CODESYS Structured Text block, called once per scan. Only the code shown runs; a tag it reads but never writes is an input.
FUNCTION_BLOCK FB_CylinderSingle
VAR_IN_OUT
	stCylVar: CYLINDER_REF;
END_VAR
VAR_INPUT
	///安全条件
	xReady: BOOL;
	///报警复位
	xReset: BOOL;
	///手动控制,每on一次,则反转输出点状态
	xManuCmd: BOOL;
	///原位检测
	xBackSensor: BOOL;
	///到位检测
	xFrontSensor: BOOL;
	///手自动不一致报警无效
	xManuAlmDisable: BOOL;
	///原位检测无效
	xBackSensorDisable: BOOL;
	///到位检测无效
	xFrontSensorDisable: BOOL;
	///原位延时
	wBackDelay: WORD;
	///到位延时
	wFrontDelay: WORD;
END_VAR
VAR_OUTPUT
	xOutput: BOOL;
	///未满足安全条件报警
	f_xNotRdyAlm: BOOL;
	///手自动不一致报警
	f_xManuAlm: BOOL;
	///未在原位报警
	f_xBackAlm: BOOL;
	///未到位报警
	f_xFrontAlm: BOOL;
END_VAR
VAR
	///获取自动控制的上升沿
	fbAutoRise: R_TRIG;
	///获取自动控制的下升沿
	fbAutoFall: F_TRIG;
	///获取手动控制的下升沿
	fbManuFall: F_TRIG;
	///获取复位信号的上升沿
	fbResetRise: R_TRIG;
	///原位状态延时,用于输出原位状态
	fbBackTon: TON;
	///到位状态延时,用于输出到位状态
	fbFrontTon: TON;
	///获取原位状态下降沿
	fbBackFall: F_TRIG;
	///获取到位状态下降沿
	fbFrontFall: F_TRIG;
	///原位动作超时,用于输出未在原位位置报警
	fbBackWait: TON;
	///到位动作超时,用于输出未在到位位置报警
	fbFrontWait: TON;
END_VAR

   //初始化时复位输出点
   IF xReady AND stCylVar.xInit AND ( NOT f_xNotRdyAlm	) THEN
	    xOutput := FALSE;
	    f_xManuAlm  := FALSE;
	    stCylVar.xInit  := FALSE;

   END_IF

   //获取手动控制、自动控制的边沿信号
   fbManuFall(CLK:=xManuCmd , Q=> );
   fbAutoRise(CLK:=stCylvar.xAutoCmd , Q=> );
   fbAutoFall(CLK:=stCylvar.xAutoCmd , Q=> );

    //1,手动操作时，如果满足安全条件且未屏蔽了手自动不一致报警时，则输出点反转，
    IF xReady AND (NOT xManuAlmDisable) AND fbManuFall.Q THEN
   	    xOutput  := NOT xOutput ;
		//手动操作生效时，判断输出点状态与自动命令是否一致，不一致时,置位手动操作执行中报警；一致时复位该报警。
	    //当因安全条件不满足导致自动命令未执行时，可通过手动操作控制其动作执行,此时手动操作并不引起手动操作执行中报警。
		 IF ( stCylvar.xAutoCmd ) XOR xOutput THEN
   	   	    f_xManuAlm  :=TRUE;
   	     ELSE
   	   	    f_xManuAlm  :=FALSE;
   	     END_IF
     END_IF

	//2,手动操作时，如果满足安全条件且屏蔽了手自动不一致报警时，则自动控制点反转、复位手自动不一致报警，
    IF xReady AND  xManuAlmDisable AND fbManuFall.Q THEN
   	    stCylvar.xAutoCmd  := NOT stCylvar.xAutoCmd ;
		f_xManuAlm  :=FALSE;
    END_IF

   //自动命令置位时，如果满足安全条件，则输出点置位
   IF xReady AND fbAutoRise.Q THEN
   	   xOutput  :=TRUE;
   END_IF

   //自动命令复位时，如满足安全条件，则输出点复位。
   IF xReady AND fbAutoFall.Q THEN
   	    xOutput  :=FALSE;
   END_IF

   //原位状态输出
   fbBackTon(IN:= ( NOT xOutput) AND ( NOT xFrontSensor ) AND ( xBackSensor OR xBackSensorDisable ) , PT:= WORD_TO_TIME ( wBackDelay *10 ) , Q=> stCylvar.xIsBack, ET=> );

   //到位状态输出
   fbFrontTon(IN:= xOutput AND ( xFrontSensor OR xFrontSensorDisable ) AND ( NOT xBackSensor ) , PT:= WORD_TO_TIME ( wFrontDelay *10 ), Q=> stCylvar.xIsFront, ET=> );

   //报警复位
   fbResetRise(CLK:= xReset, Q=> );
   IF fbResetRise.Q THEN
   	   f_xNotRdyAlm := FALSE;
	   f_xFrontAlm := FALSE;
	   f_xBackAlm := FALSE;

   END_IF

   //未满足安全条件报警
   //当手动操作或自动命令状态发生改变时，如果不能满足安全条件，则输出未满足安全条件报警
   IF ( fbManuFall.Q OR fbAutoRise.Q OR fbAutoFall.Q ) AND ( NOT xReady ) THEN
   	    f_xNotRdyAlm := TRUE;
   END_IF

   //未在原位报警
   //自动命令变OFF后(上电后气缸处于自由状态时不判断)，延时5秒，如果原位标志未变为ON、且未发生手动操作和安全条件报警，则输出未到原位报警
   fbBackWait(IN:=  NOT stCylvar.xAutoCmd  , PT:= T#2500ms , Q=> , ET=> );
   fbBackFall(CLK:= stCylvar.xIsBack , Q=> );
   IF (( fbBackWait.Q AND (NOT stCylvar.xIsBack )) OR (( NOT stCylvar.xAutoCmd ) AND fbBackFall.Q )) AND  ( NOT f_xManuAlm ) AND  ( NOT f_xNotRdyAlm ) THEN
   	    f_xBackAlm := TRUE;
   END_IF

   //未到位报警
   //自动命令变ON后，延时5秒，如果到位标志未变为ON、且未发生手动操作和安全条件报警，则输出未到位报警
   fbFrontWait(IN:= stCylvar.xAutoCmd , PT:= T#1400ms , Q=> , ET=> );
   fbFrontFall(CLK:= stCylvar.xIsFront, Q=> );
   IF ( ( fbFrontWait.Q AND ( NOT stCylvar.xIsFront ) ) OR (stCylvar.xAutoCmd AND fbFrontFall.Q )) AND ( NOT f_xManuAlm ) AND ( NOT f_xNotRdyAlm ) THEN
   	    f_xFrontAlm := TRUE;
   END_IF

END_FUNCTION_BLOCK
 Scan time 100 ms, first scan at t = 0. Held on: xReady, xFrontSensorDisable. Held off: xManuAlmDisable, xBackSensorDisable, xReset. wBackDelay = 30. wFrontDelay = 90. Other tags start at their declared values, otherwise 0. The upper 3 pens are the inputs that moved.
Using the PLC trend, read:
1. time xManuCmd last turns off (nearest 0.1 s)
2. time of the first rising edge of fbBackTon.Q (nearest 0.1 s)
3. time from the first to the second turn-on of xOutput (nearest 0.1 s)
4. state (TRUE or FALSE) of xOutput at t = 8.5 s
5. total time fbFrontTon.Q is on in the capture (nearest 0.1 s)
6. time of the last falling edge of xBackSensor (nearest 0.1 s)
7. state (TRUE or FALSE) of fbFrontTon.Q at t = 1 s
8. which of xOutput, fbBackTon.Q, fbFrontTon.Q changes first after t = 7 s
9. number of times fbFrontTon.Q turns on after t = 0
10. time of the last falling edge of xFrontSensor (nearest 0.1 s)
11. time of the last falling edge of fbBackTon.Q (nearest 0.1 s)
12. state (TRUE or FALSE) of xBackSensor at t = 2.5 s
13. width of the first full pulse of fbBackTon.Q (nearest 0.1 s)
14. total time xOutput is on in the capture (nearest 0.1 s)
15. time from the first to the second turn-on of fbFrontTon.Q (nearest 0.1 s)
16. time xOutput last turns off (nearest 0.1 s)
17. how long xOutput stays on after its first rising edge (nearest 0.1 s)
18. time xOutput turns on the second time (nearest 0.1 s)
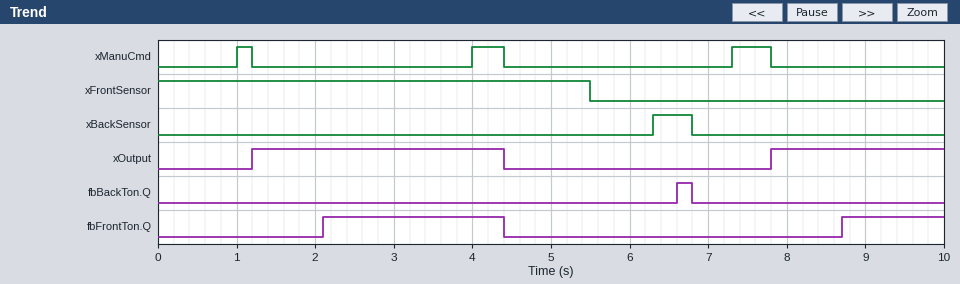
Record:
7.8 s
6.6 s
6.6 s
TRUE
3.6 s
6.8 s
FALSE
xOutput
2
5.5 s
6.8 s
FALSE
0.2 s
5.4 s
6.6 s
4.4 s
3.2 s
7.8 s
